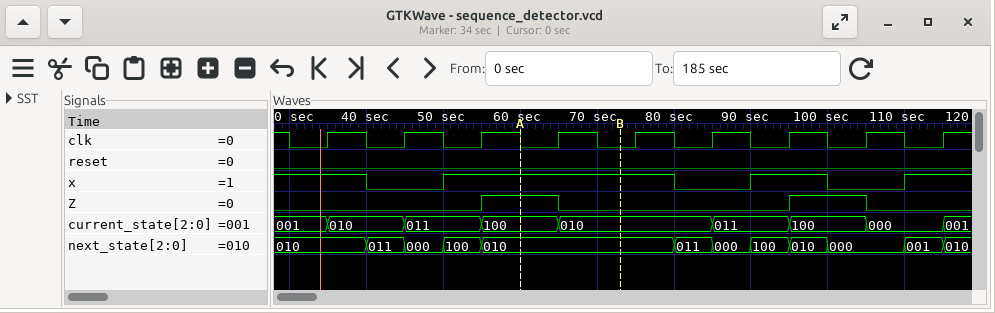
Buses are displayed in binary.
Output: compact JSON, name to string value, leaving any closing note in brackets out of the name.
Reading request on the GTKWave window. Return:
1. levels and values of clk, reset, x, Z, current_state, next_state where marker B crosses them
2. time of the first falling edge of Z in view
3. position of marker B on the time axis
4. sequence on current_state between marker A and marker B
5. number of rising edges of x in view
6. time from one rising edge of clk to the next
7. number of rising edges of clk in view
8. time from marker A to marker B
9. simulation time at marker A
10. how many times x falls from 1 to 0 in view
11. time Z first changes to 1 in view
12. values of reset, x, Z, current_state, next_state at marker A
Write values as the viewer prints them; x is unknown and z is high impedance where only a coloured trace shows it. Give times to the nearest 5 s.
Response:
{"levels and values of clk, reset, x, Z, current_state, next_state where marker B crosses them": "clk=0, reset=0, x=1, Z=0, current_state=010, next_state=010", "time of the first falling edge of Z in view": "65 s", "position of marker B on the time axis": "75 s", "sequence on current_state between marker A and marker B": "100, 010", "number of rising edges of x in view": "3", "time from one rising edge of clk to the next": "10 s", "number of rising edges of clk in view": "9", "time from marker A to marker B": "15 s", "simulation time at marker A": "60 s", "how many times x falls from 1 to 0 in view": "3", "time Z first changes to 1 in view": "55 s", "values of reset, x, Z, current_state, next_state at marker A": "reset=0, x=1, Z=1, current_state=100, next_state=010"}
